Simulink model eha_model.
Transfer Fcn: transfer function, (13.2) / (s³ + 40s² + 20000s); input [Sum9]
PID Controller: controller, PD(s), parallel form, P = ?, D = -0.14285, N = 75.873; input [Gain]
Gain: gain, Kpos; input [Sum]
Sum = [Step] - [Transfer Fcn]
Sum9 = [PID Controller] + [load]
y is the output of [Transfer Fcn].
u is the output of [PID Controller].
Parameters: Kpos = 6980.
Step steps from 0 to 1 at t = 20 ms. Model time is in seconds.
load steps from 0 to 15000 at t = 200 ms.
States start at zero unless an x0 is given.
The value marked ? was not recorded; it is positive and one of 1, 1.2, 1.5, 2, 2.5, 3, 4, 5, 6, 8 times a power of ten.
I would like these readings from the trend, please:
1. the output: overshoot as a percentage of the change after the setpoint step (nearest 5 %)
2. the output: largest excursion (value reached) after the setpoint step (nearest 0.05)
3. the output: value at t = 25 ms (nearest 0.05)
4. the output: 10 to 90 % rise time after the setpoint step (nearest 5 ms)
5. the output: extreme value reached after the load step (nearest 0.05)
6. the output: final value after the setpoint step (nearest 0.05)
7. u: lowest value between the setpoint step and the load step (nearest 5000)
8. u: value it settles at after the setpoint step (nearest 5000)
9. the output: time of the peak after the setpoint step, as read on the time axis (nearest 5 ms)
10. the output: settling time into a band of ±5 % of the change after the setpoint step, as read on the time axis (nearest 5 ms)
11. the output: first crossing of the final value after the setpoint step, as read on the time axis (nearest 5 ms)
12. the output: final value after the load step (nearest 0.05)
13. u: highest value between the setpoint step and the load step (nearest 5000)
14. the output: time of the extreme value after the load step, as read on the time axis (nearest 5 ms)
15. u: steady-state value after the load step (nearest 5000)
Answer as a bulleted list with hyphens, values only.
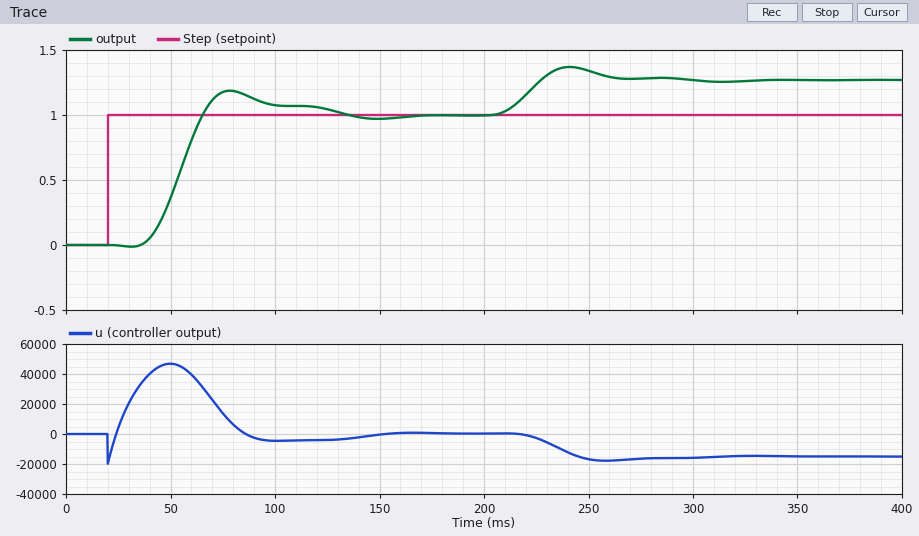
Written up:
- 20 %
- 1.20
- 0.00
- 20 ms
- 1.35
- 1.00
- -20000
- 0
- 80 ms
- 125 ms
- 65 ms
- 1.25
- 45000
- 240 ms
- -15000
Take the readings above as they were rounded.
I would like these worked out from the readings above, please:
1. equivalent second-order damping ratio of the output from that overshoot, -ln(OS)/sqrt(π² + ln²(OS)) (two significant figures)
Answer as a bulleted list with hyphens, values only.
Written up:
- 0.46
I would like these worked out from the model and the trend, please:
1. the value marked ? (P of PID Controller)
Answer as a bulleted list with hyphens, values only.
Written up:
- 8
